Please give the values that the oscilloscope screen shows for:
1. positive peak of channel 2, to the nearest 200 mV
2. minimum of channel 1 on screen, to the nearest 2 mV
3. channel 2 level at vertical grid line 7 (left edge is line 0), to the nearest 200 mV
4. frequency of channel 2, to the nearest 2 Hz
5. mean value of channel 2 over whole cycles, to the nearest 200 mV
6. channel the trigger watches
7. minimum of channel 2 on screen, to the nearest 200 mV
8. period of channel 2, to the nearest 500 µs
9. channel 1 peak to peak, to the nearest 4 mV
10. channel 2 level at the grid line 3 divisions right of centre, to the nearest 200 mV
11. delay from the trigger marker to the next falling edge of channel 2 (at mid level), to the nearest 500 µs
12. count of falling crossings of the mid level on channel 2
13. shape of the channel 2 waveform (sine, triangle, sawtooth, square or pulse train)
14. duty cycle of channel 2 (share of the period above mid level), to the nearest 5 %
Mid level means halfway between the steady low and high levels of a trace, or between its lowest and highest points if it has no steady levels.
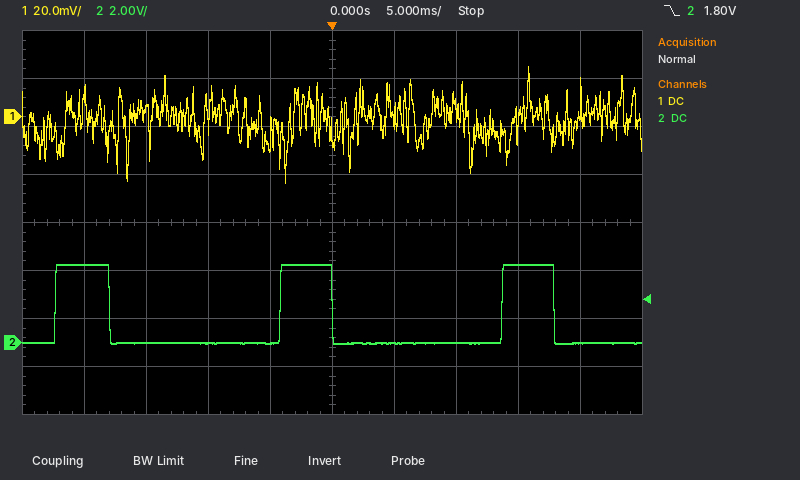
3.2 V
-28 mV
0.0 V
56 Hz
800 mV
channel 2
0.0 V
18.0 ms
48 mV
3.2 V
18.0 ms
3
pulse train
25 %
